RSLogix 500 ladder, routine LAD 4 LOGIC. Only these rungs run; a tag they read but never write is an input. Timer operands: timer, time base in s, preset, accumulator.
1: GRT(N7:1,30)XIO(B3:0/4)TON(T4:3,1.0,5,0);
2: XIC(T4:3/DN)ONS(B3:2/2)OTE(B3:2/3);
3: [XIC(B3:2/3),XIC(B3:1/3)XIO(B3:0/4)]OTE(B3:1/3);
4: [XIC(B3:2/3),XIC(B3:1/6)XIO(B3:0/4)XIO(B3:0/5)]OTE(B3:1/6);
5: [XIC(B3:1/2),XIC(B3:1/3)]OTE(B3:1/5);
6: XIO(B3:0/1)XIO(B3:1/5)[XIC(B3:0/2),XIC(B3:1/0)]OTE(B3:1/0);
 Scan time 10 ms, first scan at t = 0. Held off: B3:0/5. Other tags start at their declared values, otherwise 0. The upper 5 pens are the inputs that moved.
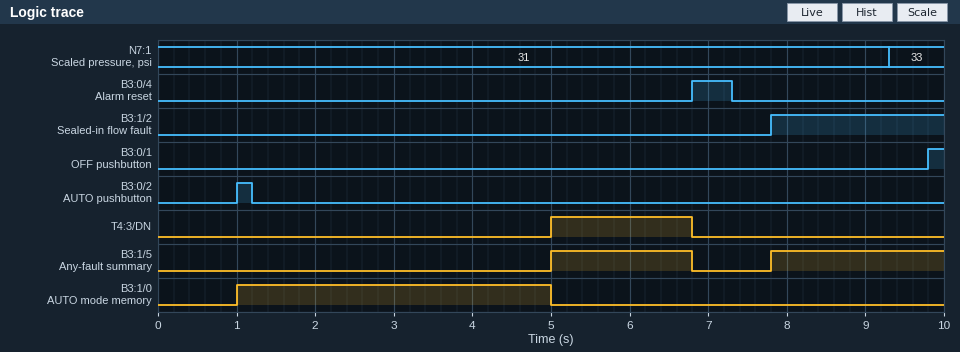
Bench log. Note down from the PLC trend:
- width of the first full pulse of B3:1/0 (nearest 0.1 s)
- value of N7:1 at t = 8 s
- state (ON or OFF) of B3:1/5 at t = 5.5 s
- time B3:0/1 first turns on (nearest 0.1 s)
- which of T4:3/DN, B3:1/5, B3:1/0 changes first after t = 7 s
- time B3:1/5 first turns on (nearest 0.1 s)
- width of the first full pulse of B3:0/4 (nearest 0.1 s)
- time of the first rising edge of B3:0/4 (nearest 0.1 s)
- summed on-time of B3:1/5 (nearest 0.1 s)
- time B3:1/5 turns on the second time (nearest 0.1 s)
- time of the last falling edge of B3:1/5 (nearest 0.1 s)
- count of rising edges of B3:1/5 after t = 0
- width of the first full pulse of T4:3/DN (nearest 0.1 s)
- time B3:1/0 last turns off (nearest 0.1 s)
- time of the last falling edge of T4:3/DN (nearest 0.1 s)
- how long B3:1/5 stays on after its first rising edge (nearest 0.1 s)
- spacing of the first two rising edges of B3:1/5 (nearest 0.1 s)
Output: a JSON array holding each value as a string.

["4.0 s", "31", "ON", "9.8 s", "B3:1/5", "5.0 s", "0.5 s", "6.8 s", "4.0 s", "7.8 s", "6.8 s", "2", "1.8 s", "5.0 s", "6.8 s", "1.8 s", "2.8 s"]
